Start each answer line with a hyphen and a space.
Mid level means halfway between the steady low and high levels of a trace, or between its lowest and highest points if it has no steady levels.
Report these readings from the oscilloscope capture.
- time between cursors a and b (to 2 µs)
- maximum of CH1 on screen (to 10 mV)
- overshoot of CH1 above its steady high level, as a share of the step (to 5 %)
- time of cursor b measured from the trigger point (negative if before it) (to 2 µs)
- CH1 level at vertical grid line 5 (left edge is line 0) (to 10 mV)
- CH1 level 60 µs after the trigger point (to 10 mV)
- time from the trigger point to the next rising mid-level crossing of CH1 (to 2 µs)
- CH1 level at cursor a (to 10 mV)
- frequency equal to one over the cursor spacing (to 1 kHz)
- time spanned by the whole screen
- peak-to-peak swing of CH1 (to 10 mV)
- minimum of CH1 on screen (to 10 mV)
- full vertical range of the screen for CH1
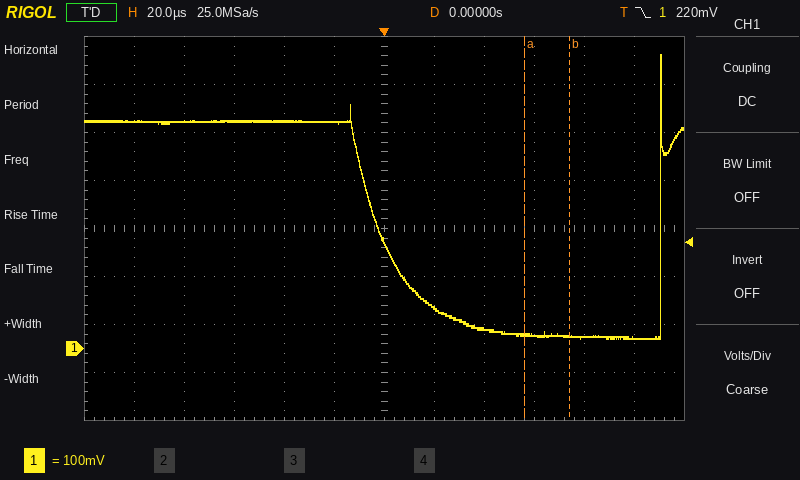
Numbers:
- 18 µs
- 610 mV
- 30 %
- +74 µs
- 470 mV
- 30 mV
- 110 µs
- 30 mV
- 56 kHz
- 240 µs
- 590 mV
- 20 mV
- 800 mV
